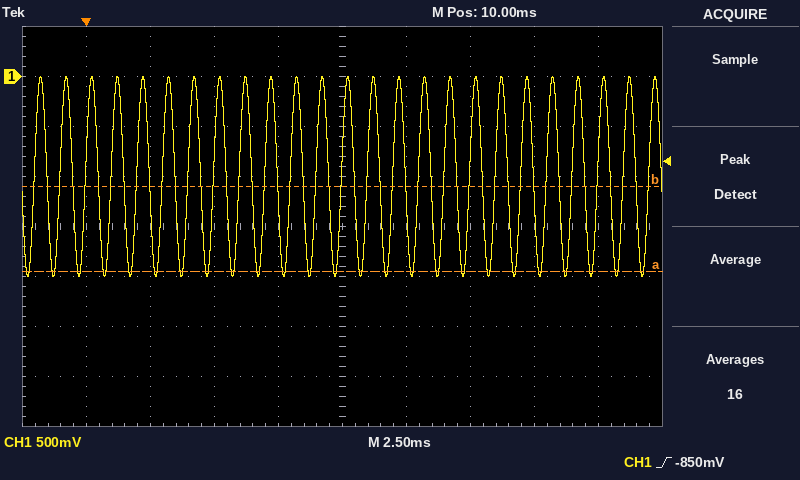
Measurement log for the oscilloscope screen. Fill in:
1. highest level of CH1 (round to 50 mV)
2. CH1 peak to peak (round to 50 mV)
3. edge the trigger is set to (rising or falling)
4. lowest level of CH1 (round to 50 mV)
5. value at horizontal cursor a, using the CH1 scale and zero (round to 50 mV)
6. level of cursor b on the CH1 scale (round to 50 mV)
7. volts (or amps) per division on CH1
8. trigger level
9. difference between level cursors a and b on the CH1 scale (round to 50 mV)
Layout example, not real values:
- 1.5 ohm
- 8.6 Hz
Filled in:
- 0 mV
- 2.00 V
- rising
- -2.00 V
- -1.95 V
- -1.10 V
- 500 mV
- -850 mV
- 850 mV
